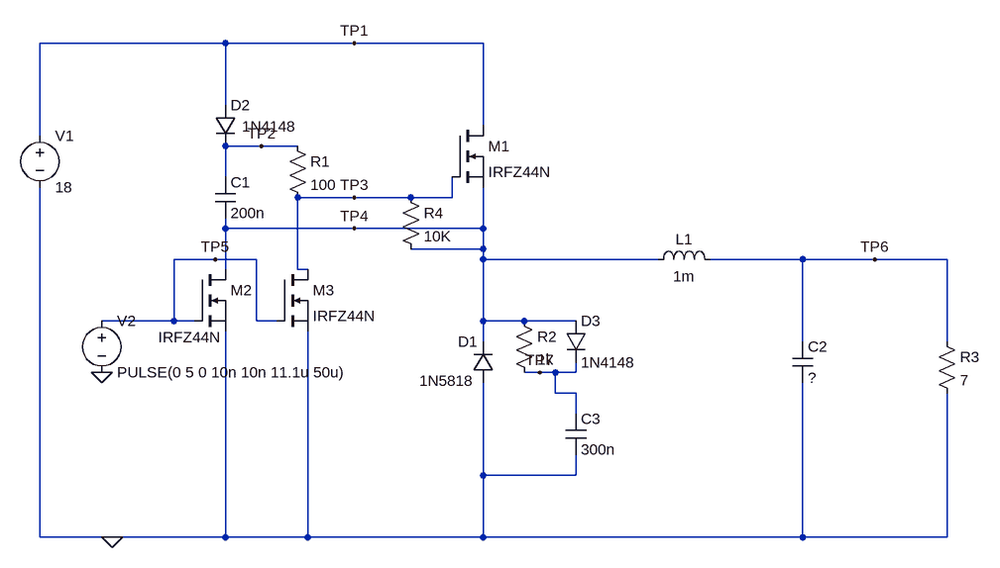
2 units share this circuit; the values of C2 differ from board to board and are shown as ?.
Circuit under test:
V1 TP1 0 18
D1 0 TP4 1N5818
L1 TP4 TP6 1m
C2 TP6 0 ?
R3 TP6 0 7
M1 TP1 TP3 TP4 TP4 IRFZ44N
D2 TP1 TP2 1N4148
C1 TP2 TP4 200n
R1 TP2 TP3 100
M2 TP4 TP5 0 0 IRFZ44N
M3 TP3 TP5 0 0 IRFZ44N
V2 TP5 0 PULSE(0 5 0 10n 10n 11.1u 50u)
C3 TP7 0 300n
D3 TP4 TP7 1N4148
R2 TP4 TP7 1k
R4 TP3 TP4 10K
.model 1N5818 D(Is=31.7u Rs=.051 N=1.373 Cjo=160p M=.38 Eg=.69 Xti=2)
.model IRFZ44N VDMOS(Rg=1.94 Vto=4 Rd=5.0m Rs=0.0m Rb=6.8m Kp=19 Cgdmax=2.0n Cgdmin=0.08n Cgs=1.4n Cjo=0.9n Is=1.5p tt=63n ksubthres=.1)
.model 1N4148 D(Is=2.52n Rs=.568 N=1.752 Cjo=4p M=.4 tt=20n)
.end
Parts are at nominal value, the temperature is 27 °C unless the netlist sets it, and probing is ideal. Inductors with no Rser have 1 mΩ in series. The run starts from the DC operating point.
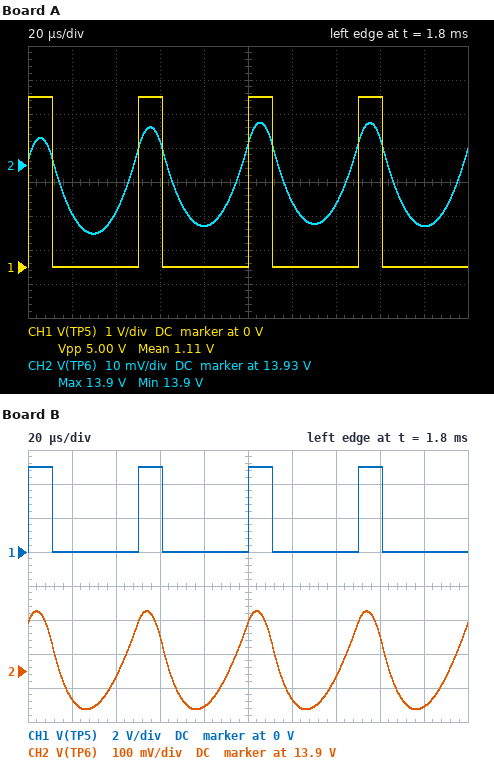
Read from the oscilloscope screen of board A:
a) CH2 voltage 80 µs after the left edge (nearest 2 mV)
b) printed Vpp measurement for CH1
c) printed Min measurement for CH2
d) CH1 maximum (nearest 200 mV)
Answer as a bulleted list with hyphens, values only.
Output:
- 13.912 V
- 5.00 V
- 13.9 V
- 5.0 V
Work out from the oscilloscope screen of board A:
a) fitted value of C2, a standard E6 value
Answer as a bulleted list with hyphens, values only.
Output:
- 33 µF
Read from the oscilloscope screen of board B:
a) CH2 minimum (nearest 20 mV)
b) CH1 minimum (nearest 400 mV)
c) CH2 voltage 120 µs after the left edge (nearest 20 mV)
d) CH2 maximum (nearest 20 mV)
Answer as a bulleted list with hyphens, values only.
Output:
- 13.78 V
- 0 V
- 13.82 V
- 14.08 V
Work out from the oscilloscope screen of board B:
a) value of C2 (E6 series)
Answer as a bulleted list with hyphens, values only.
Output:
- 3.3 µF
